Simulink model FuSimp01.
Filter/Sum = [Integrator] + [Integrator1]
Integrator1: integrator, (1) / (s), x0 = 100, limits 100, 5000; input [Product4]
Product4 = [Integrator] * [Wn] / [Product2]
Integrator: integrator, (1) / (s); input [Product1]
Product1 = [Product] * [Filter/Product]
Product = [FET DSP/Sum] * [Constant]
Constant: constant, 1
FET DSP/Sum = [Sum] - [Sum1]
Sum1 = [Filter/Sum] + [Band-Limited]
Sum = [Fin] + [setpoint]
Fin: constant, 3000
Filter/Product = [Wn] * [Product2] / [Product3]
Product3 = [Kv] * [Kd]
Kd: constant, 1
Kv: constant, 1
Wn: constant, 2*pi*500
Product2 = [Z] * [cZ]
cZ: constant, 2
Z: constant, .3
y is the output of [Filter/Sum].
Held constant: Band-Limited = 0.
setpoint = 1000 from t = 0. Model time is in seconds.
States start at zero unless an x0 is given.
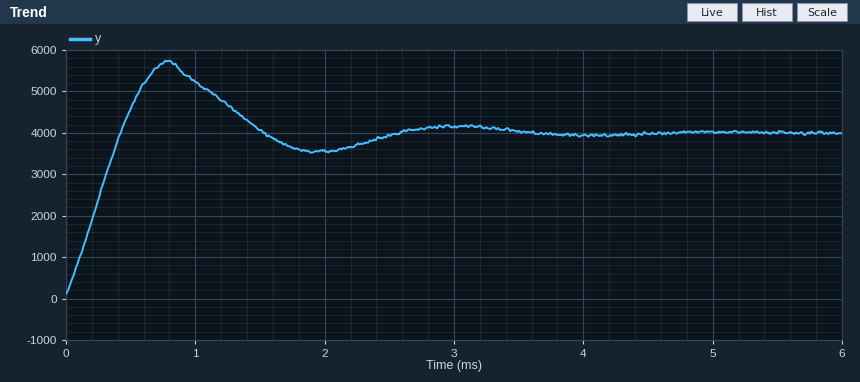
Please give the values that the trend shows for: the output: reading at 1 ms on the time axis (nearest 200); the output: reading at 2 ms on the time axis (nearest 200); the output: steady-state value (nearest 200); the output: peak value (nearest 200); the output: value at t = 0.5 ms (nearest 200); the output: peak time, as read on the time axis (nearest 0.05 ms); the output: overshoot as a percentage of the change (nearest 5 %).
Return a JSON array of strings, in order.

["5200", "3600", "4000", "5800", "4600", "0.80 ms", "45 %"]
